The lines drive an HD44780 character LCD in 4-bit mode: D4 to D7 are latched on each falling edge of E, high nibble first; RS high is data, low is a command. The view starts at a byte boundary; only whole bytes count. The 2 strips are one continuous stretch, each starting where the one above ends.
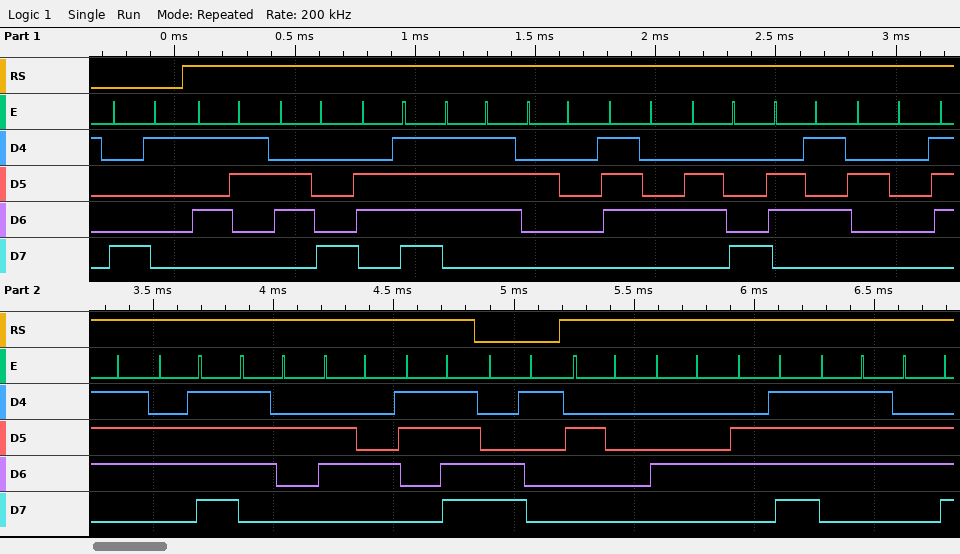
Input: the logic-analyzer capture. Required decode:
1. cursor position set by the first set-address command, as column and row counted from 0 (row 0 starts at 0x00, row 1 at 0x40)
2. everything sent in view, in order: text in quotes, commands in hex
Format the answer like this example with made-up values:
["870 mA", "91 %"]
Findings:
["column 1, row 0", "0x81 \"Show the word?\" 0xC1 \" Down\""]
